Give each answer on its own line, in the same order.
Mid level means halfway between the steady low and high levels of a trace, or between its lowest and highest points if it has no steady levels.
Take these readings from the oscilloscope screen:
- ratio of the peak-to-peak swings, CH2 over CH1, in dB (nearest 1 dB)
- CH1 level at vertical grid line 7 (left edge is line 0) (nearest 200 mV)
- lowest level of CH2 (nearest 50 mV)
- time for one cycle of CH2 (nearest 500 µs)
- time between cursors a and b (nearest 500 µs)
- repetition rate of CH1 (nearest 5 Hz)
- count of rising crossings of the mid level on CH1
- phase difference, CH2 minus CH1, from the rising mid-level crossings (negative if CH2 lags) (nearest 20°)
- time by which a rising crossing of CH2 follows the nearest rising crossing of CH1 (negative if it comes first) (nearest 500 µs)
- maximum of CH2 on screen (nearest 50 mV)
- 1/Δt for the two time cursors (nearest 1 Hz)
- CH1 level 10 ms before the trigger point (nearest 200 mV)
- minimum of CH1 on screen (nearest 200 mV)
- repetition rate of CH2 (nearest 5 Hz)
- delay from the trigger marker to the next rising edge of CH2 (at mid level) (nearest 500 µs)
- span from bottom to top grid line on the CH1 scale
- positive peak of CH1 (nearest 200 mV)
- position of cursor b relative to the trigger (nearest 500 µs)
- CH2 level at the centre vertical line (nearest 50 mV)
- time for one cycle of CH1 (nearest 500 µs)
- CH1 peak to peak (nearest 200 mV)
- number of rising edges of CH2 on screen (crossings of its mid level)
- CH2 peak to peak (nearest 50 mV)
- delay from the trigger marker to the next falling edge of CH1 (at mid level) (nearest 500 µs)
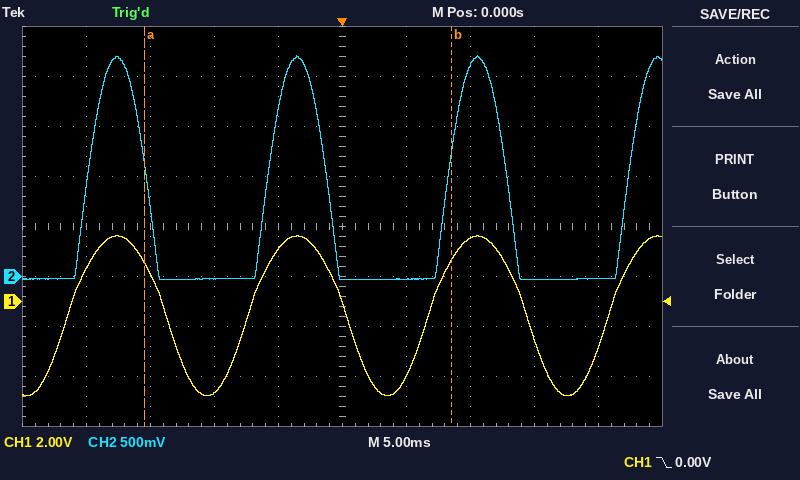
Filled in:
-9 dB
2.6 V
-50 mV
14.0 ms
24.0 ms
70 Hz
4
-40°
+1.5 ms
2.20 V
42 Hz
-3.6 V
-3.8 V
70 Hz
8.5 ms
16 V
2.6 V
+8.5 ms
0 mV
14.0 ms
6.4 V
4
2.25 V
500 µs
